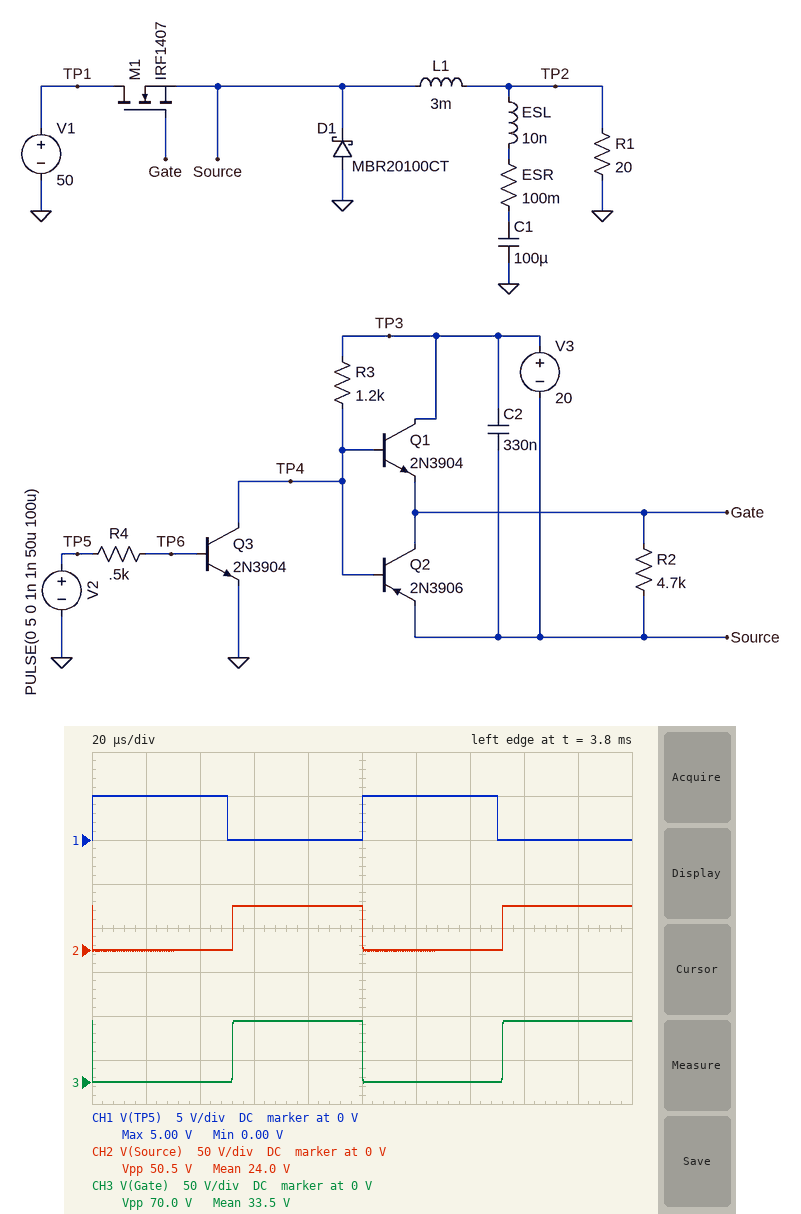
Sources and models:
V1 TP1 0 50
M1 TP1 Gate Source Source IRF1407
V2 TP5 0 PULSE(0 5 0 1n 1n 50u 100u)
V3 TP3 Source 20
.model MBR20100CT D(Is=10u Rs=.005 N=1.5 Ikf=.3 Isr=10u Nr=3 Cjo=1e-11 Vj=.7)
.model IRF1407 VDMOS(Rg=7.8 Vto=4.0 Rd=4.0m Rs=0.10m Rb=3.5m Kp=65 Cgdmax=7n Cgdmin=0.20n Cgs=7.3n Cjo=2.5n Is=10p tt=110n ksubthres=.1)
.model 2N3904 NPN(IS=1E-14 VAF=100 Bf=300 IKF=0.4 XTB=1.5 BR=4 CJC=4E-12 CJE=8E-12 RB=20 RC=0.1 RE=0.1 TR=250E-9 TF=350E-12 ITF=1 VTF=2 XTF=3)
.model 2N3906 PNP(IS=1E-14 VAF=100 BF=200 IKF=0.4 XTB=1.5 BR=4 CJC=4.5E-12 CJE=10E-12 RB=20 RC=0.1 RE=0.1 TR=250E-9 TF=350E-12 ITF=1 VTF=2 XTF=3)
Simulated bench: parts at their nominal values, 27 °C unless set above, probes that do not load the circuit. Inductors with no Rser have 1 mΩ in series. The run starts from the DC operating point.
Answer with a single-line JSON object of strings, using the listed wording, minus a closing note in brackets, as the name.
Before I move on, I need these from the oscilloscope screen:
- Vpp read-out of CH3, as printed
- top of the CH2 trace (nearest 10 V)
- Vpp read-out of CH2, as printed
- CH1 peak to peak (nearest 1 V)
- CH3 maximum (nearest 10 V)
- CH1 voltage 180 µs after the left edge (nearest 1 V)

{"Vpp read-out of CH3, as printed": "70.0 V", "top of the CH2 trace": "50 V", "Vpp read-out of CH2, as printed": "50.5 V", "CH1 peak to peak": "5 V", "CH3 maximum": "70 V", "CH1 voltage 180 µs after the left edge": "0 V"}
